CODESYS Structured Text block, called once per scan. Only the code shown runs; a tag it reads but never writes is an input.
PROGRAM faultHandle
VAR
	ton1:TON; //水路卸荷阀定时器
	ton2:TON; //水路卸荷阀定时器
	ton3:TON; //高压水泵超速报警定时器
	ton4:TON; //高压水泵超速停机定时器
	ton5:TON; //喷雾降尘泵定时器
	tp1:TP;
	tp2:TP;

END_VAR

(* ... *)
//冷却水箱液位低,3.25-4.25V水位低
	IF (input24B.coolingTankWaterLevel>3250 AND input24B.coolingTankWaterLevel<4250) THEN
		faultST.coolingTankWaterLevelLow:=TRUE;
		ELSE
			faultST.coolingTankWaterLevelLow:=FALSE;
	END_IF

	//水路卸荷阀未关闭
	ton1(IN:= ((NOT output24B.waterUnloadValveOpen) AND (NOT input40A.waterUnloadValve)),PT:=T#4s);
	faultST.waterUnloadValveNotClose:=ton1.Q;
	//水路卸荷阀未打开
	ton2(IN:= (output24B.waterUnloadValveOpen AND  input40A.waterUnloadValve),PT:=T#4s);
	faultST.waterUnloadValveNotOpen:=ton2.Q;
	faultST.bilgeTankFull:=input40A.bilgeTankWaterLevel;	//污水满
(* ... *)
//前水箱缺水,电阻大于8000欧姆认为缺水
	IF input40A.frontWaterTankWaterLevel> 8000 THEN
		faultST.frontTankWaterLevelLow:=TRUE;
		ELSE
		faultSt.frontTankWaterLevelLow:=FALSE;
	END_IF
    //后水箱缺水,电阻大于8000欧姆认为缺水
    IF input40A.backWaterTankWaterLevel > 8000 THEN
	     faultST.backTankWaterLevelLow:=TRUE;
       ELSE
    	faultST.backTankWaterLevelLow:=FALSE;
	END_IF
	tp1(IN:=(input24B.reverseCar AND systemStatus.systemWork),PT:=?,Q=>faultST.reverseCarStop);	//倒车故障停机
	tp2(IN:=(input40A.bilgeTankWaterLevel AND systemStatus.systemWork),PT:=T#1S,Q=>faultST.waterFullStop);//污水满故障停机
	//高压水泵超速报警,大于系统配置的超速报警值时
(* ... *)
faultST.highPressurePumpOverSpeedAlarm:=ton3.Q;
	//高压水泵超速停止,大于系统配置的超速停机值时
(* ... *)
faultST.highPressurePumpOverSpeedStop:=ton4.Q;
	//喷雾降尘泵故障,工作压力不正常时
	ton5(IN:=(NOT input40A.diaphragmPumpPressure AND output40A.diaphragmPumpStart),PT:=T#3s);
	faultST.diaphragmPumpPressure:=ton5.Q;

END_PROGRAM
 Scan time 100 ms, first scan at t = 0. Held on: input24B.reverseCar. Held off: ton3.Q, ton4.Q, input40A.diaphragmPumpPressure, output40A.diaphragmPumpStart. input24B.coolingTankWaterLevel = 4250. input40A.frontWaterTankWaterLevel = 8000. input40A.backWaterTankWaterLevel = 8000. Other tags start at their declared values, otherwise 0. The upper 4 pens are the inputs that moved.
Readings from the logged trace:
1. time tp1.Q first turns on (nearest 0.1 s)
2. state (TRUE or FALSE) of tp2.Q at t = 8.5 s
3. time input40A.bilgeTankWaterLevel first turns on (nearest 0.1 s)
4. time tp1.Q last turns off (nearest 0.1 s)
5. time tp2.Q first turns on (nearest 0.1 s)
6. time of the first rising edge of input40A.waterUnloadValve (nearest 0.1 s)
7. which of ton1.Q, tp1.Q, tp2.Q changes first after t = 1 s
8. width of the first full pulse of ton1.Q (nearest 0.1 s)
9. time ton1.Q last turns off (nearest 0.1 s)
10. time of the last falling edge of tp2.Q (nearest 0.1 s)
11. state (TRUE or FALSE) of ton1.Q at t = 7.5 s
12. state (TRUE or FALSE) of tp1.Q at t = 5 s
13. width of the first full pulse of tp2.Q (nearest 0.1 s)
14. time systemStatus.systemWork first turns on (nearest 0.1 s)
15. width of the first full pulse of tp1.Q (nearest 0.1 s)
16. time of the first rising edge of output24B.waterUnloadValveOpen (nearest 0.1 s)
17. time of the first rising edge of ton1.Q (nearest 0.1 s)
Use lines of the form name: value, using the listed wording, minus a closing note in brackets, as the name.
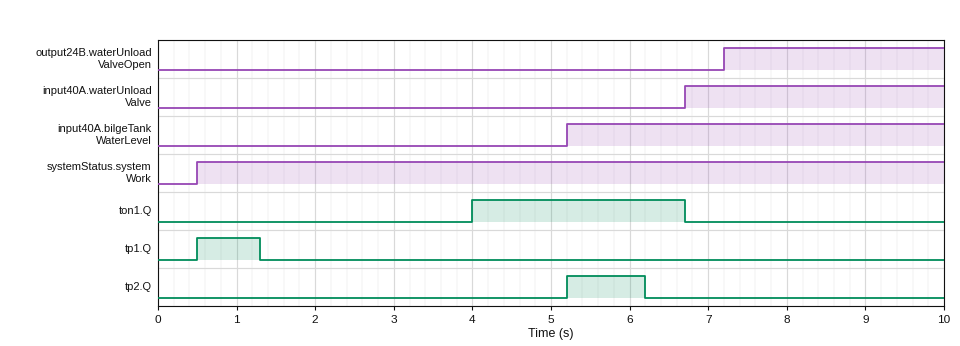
time tp1.Q first turns on: 0.5 s
state (TRUE or FALSE) of tp2.Q at t = 8.5 s: FALSE
time input40A.bilgeTankWaterLevel first turns on: 5.2 s
time tp1.Q last turns off: 1.3 s
time tp2.Q first turns on: 5.2 s
time of the first rising edge of input40A.waterUnloadValve: 6.7 s
which of ton1.Q, tp1.Q, tp2.Q changes first after t = 1 s: tp1.Q
width of the first full pulse of ton1.Q: 2.7 s
time ton1.Q last turns off: 6.7 s
time of the last falling edge of tp2.Q: 6.2 s
state (TRUE or FALSE) of ton1.Q at t = 7.5 s: FALSE
state (TRUE or FALSE) of tp1.Q at t = 5 s: FALSE
width of the first full pulse of tp2.Q: 1.0 s
time systemStatus.systemWork first turns on: 0.5 s
width of the first full pulse of tp1.Q: 0.8 s
time of the first rising edge of output24B.waterUnloadValveOpen: 7.2 s
time of the first rising edge of ton1.Q: 4.0 s
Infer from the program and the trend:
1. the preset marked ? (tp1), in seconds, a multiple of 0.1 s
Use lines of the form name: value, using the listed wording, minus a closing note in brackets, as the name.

the preset marked ? (tp1), in seconds, a multiple of 0.1 s: 0.8 s
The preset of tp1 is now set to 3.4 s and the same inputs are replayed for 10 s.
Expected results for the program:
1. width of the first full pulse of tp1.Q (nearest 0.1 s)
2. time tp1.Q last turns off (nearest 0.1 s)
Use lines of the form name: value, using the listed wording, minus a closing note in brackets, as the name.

width of the first full pulse of tp1.Q: 3.4 s
time tp1.Q last turns off: 3.9 s
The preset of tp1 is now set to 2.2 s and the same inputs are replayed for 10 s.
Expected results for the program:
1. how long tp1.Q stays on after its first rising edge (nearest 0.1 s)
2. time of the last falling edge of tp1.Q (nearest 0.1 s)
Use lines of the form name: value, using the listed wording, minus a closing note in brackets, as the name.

how long tp1.Q stays on after its first rising edge: 2.2 s
time of the last falling edge of tp1.Q: 2.7 s
